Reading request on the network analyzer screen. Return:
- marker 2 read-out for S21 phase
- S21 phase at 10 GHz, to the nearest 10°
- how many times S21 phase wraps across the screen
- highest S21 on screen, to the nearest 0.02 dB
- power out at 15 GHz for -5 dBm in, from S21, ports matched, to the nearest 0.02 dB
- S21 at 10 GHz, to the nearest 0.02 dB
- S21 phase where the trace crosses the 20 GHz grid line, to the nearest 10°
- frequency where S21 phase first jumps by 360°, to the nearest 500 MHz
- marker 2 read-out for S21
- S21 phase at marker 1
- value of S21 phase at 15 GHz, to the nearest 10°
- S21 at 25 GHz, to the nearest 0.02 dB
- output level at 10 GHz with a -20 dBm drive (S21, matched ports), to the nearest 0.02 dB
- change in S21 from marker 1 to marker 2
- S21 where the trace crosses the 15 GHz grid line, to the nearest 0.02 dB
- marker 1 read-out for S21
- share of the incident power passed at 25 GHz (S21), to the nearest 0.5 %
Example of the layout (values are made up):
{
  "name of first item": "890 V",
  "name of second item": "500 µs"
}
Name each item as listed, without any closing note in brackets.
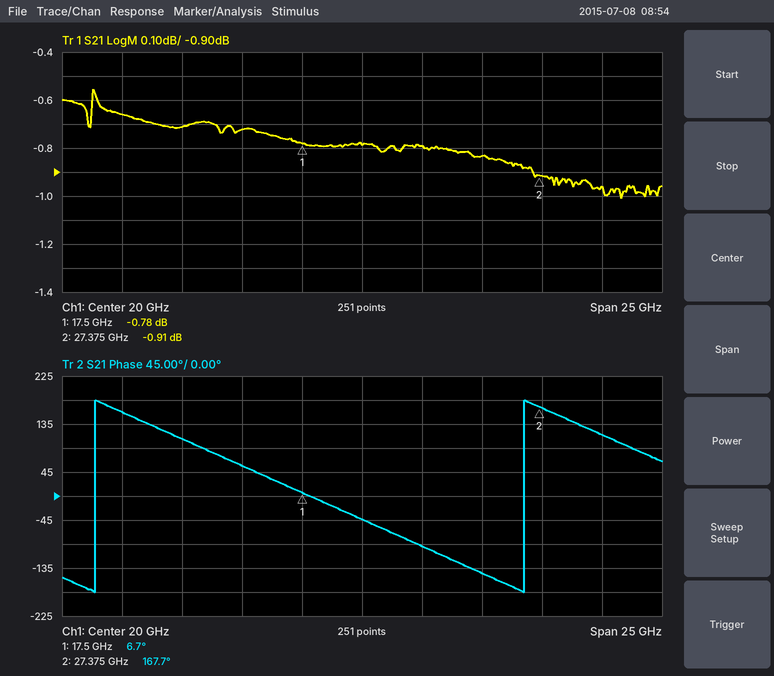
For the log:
{
  "marker 2 read-out for S21 phase": "167.7°",
  "S21 phase at 10 GHz, to the nearest 10°": "160°",
  "how many times S21 phase wraps across the screen": "2",
  "highest S21 on screen, to the nearest 0.02 dB": "-0.56 dB",
  "power out at 15 GHz for -5 dBm in, from S21, ports matched, to the nearest 0.02 dB": "-5.72 dBm",
  "S21 at 10 GHz, to the nearest 0.02 dB": "-0.66 dB",
  "S21 phase where the trace crosses the 20 GHz grid line, to the nearest 10°": "-40°",
  "frequency where S21 phase first jumps by 360°, to the nearest 500 MHz": "9.0 GHz",
  "marker 2 read-out for S21": "-0.91 dB",
  "S21 phase at marker 1": "6.7°",
  "value of S21 phase at 15 GHz, to the nearest 10°": "60°",
  "S21 at 25 GHz, to the nearest 0.02 dB": "-0.84 dB",
  "output level at 10 GHz with a -20 dBm drive (S21, matched ports), to the nearest 0.02 dB": "-20.66 dBm",
  "change in S21 from marker 1 to marker 2": "-0.13 dB",
  "S21 where the trace crosses the 15 GHz grid line, to the nearest 0.02 dB": "-0.72 dB",
  "marker 1 read-out for S21": "-0.78 dB",
  "share of the incident power passed at 25 GHz (S21), to the nearest 0.5 %": "82.5 %"
}
